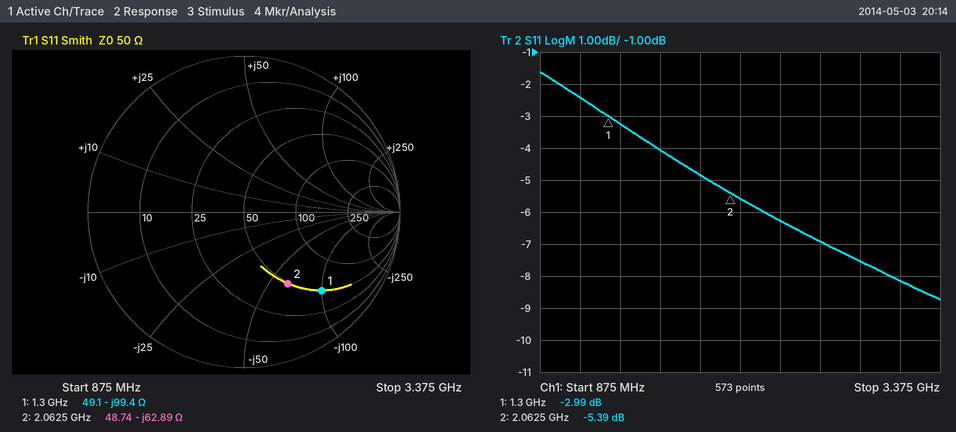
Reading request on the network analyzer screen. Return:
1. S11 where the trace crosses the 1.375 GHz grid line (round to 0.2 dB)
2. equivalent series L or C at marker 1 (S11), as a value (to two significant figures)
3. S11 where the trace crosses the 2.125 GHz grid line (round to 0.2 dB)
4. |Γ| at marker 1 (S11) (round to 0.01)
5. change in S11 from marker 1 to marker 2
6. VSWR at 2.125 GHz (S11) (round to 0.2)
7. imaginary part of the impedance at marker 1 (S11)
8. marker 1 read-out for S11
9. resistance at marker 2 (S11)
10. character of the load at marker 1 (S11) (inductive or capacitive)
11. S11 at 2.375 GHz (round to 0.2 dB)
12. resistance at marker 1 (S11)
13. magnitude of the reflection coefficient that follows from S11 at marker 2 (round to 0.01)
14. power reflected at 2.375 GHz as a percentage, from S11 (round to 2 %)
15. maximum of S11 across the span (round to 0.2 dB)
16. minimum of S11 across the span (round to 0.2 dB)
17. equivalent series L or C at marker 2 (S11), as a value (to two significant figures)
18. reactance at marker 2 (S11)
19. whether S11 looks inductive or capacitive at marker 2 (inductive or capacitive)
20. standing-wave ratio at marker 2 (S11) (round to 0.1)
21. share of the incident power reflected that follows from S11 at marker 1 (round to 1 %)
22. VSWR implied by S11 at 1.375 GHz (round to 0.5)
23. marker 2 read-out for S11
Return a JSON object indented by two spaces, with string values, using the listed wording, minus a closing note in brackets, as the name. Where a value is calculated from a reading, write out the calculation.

{
  "S11 where the trace crosses the 1.375 GHz grid line": "-3.2 dB",
  "equivalent series L or C at marker 1 (S11), as a value": "C = 1/(2π × 1.3 GHz × 99.4 Ω) ≈ 1.2 pF",
  "S11 where the trace crosses the 2.125 GHz grid line": "-5.6 dB",
  "|Γ| at marker 1 (S11)": "0.71",
  "change in S11 from marker 1 to marker 2": "-5.39 − (-2.99) = -2.40 dB",
  "VSWR at 2.125 GHz (S11)": "|Γ| = 10^(-5.6/20) = 0.5248; VSWR = (1 + 0.5248)/(1 − 0.5248) ≈ 3.2",
  "imaginary part of the impedance at marker 1": "-99.4 Ω",
  "marker 1 read-out for S11": "-2.99 dB",
  "resistance at marker 2": "48.74 Ω",
  "character of the load at marker 1 (S11)": "capacitive",
  "S11 at 2.375 GHz": "-6.2 dB",
  "resistance at marker 1": "49.1 Ω",
  "magnitude of the reflection coefficient that follows from S11 at marker 2": "10^(-5.39/20) ≈ 0.54",
  "power reflected at 2.375 GHz as a percentage, from S11": "10^(-6.2/10) ≈ 24 %",
  "maximum of S11 across the span": "-1.6 dB",
  "minimum of S11 across the span": "-8.8 dB",
  "equivalent series L or C at marker 2 (S11), as a value": "C = 1/(2π × 2.0625 GHz × 62.89 Ω) ≈ 1.2 pF",
  "reactance at marker 2": "-62.89 Ω",
  "whether S11 looks inductive or capacitive at marker 2": "capacitive",
  "standing-wave ratio at marker 2 (S11)": "3.3",
  "share of the incident power reflected that follows from S11 at marker 1": "10^(-2.99/10) ≈ 50 %",
  "VSWR implied by S11 at 1.375 GHz": "|Γ| = 10^(-3.2/20) = 0.6918; VSWR = (1 + 0.6918)/(1 − 0.6918) ≈ 5.5",
  "marker 2 read-out for S11": "-5.39 dB"
}
